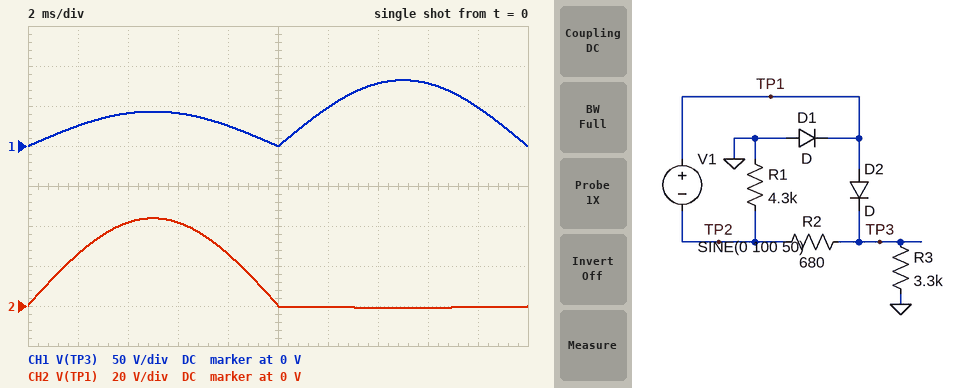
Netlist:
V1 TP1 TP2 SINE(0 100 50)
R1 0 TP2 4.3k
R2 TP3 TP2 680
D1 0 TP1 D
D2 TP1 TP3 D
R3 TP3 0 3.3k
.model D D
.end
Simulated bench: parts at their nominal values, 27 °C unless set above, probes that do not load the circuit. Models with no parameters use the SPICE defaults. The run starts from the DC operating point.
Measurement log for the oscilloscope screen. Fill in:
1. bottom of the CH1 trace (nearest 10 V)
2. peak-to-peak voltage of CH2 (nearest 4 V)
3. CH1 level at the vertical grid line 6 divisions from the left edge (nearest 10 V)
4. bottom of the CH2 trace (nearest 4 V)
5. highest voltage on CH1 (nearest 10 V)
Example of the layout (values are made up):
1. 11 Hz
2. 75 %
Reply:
1. 0 V
2. 44 V
3. 50 V
4. 0 V
5. 80 V
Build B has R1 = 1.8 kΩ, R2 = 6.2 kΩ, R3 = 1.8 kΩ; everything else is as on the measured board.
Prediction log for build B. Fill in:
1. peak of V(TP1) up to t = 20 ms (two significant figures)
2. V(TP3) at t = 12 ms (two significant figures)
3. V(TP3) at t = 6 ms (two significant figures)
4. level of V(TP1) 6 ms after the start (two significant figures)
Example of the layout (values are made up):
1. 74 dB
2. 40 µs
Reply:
1. 50 V
2. 13 V
3. 47 V
4. 48 V
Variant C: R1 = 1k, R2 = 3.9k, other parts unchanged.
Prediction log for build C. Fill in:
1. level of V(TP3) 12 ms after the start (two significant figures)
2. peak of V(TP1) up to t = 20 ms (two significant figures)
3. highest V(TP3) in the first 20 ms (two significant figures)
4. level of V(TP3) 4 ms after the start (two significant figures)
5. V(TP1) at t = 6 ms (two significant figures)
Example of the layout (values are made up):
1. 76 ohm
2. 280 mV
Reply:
1. 27 V
2. 77 V
3. 76 V
4. 72 V
5. 73 V
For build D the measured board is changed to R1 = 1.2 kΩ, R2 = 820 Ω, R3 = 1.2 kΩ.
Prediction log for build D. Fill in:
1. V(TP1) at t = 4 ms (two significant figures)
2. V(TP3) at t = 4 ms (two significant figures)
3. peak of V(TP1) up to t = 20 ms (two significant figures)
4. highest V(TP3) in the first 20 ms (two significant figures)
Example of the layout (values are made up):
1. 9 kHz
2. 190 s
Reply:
1. 48 V
2. 47 V
3. 50 V
4. 59 V
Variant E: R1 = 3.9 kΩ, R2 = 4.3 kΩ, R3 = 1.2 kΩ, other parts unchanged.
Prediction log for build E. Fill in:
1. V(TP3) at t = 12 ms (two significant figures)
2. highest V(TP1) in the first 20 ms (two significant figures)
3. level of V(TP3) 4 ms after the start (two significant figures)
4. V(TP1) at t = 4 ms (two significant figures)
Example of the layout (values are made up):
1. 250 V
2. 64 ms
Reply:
1. 13 V
2. 24 V
3. 22 V
4. 23 V
